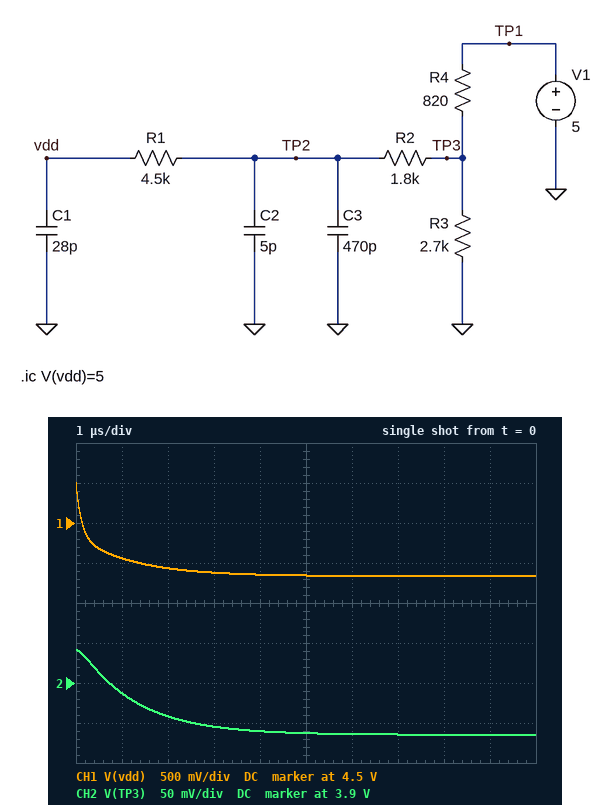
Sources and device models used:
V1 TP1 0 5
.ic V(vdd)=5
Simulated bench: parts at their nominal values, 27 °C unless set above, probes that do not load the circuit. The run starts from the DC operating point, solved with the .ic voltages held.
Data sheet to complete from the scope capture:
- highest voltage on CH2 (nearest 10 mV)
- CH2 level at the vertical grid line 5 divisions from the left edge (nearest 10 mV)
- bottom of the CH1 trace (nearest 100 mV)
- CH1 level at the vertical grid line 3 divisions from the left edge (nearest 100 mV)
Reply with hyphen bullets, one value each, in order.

- 3.94 V
- 3.84 V
- 3.8 V
- 3.9 V
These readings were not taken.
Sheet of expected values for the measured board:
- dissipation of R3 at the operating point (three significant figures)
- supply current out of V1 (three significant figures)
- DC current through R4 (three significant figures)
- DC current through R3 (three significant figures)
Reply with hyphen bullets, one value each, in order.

- 5.45 mW
- 1.42 mA
- 1.42 mA
- 1.42 mA
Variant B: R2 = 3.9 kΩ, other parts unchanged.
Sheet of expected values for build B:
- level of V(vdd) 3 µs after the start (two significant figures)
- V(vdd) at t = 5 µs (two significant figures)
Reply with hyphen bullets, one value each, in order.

- 4.0 V
- 3.9 V
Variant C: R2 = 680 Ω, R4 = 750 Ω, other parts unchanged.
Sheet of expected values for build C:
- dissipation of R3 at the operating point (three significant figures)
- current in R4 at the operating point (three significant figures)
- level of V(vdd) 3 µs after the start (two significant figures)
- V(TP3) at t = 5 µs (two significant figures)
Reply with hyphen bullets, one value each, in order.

- 5.67 mW
- 1.45 mA
- 3.9 V
- 3.9 V
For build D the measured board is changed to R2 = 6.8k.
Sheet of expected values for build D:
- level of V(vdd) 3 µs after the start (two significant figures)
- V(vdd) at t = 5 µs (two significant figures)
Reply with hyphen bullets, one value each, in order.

- 4.2 V
- 4.0 V
